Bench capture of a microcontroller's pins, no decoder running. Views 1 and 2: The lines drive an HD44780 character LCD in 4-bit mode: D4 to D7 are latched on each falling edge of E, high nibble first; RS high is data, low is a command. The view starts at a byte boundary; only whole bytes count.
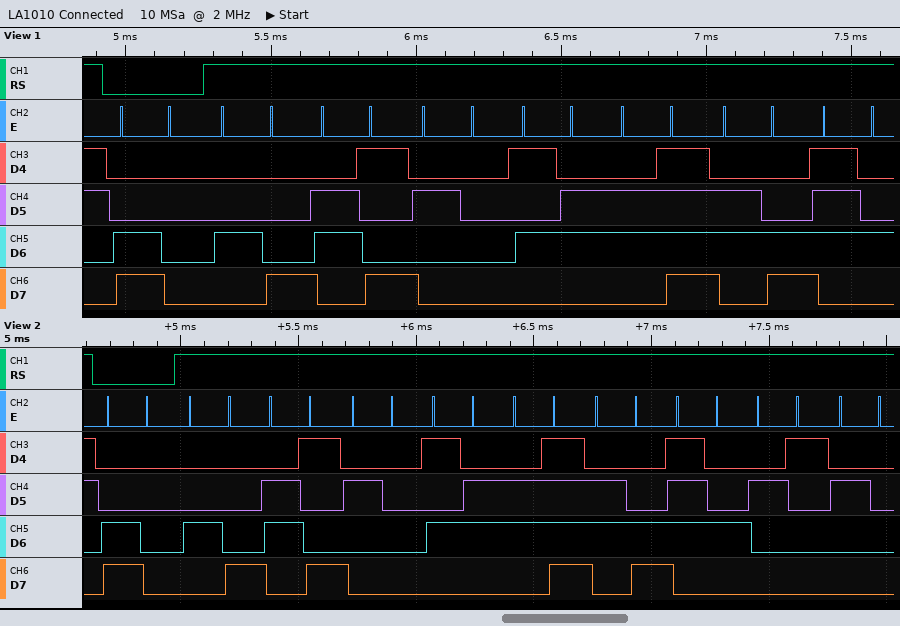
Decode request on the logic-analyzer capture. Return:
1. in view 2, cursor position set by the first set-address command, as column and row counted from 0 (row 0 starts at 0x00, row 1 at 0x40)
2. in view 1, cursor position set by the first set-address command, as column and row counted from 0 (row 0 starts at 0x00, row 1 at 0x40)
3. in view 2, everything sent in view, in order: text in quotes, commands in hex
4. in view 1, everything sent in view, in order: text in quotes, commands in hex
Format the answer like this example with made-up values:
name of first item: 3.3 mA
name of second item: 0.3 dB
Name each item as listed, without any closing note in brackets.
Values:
in view 2, cursor position set by the first set-address command, as column and row counted from 0: column 0, row 1
in view 1, cursor position set by the first set-address command, as column and row counted from 0: column 0, row 1
in view 2, everything sent in view, in order: text in quotes, commands in hex: 0xC0 "Hi Volt! "
in view 1, everything sent in view, in order: text in quotes, commands in hex: 0xC0 "Hi Volt"
